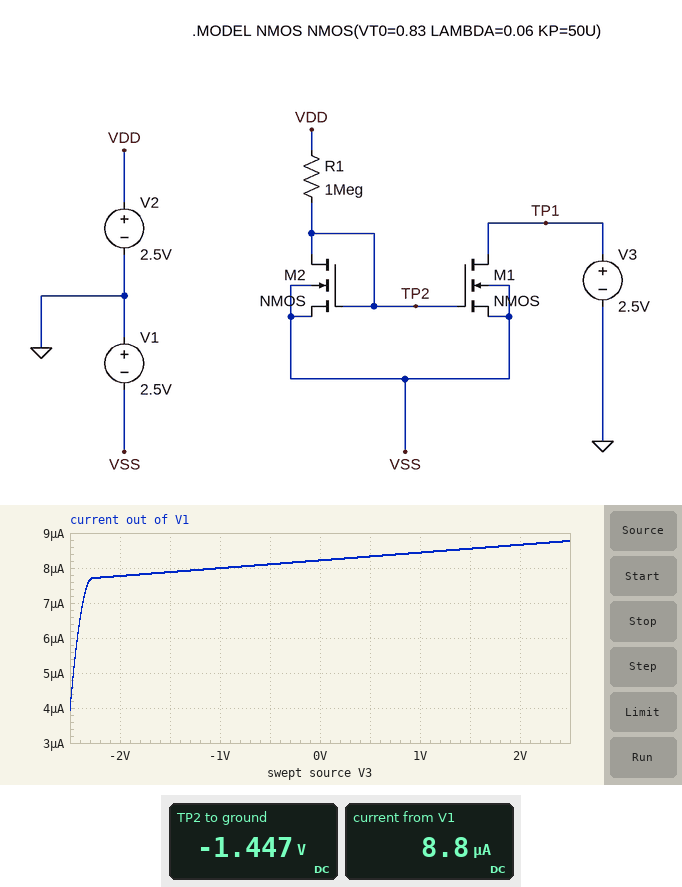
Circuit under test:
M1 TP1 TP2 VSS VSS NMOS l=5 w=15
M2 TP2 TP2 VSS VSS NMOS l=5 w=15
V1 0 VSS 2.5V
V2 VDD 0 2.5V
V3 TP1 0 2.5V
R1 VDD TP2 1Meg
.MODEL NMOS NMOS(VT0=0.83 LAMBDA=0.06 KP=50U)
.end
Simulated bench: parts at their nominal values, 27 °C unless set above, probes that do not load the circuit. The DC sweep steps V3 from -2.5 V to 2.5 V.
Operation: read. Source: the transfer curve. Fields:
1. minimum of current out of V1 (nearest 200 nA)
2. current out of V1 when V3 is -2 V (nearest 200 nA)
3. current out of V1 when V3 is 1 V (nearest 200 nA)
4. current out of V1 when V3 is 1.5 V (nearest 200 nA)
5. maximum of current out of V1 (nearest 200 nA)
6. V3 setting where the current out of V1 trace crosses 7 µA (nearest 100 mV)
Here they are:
4.0 µA
7.8 µA
8.4 µA
8.6 µA
8.8 µA
-2.4 V
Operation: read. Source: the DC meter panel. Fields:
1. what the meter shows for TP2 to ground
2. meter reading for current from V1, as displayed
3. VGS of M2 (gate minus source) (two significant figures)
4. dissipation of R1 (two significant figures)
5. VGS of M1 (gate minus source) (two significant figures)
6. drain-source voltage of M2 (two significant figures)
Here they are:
-1.447 V
8.8 µA
1.1 V
16 µW
1.1 V
1.1 V
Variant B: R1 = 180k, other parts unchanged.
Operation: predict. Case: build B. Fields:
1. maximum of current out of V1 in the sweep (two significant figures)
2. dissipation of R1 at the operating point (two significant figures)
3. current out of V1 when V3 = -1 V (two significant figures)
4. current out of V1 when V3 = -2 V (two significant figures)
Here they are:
45 µA
75 µW
41 µA
40 µA
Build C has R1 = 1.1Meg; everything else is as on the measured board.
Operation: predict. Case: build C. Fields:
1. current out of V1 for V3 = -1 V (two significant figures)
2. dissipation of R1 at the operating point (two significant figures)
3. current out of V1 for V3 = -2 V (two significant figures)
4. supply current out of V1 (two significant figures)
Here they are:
7.3 µA
14 µW
7.1 µA
8.0 µA
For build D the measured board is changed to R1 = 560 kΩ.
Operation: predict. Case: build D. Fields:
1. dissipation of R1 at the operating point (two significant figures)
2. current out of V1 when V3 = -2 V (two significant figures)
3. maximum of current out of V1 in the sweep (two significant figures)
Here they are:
27 µW
14 µA
15 µA
